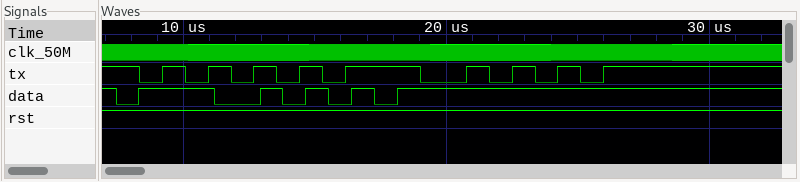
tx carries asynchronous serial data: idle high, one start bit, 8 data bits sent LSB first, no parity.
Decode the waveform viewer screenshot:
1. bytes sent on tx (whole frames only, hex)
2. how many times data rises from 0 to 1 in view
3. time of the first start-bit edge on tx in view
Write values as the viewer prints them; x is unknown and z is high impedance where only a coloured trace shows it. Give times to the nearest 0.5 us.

55, AA
5
8.5 us
